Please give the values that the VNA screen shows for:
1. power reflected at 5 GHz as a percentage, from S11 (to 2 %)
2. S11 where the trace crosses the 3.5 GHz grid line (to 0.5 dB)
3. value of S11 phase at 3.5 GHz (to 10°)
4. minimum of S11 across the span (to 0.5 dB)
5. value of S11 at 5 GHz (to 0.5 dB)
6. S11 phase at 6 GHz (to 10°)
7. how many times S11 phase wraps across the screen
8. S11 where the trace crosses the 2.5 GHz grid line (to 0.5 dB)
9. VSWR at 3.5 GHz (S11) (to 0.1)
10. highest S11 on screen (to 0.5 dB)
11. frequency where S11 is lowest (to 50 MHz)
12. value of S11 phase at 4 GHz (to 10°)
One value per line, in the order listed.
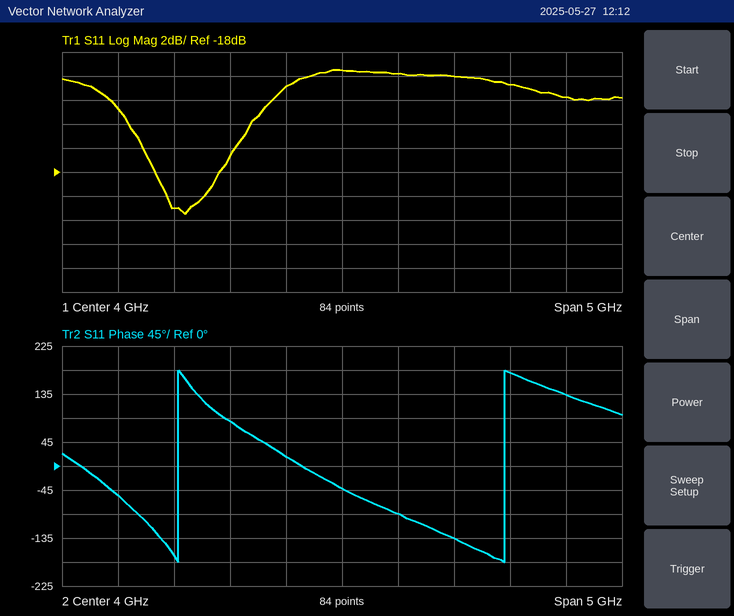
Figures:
10 %
-11.0 dB
20°
-21.5 dB
-10.0 dB
130°
2
-21.0 dB
1.8
-9.5 dB
2.60 GHz
-40°
